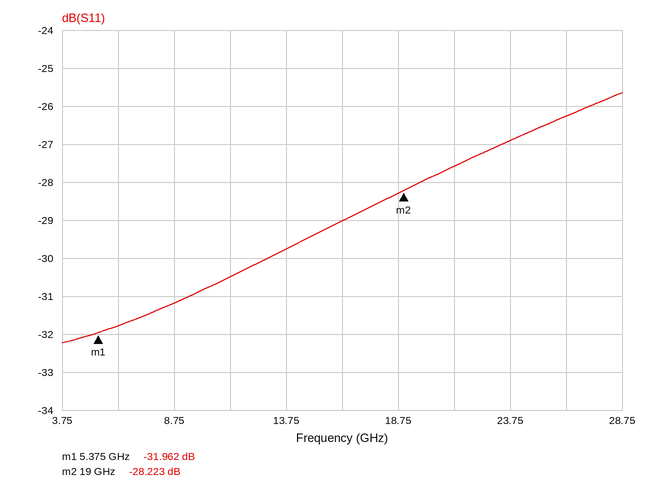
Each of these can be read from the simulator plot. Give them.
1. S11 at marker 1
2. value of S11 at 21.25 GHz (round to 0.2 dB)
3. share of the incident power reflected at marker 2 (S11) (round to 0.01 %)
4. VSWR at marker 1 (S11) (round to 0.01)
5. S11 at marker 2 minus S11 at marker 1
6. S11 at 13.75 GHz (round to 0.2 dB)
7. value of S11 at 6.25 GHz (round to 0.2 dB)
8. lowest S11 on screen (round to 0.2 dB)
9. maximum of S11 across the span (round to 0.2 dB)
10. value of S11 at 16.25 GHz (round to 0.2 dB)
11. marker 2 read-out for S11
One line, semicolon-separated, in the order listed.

-31.962 dB; -27.6 dB; 0.15 %; 1.05; 3.739 dB; -29.8 dB; -31.8 dB; -32.2 dB; -25.6 dB; -29.0 dB; -28.223 dB
